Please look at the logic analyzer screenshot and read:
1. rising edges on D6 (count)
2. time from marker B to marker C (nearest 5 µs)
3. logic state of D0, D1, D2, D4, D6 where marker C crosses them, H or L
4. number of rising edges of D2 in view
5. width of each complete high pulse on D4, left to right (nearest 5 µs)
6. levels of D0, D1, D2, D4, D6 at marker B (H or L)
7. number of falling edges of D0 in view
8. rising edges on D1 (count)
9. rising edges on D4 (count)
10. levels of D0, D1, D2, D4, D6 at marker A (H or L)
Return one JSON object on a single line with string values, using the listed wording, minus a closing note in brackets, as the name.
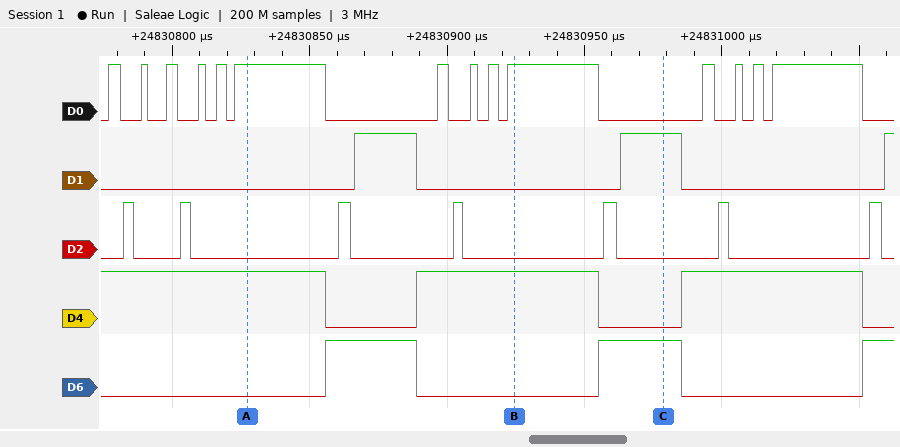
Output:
{"rising edges on D6": "3", "time from marker B to marker C": "55 µs", "logic state of D0, D1, D2, D4, D6 where marker C crosses them, H or L": "D0=L, D1=H, D2=L, D4=L, D6=H", "number of rising edges of D2 in view": "7", "width of each complete high pulse on D4, left to right": "65 µs, 65 µs", "levels of D0, D1, D2, D4, D6 at marker B": "D0=H, D1=L, D2=L, D4=H, D6=L", "number of falling edges of D0 in view": "14", "rising edges on D1": "3", "rising edges on D4": "2", "levels of D0, D1, D2, D4, D6 at marker A": "D0=H, D1=L, D2=L, D4=H, D6=L"}
